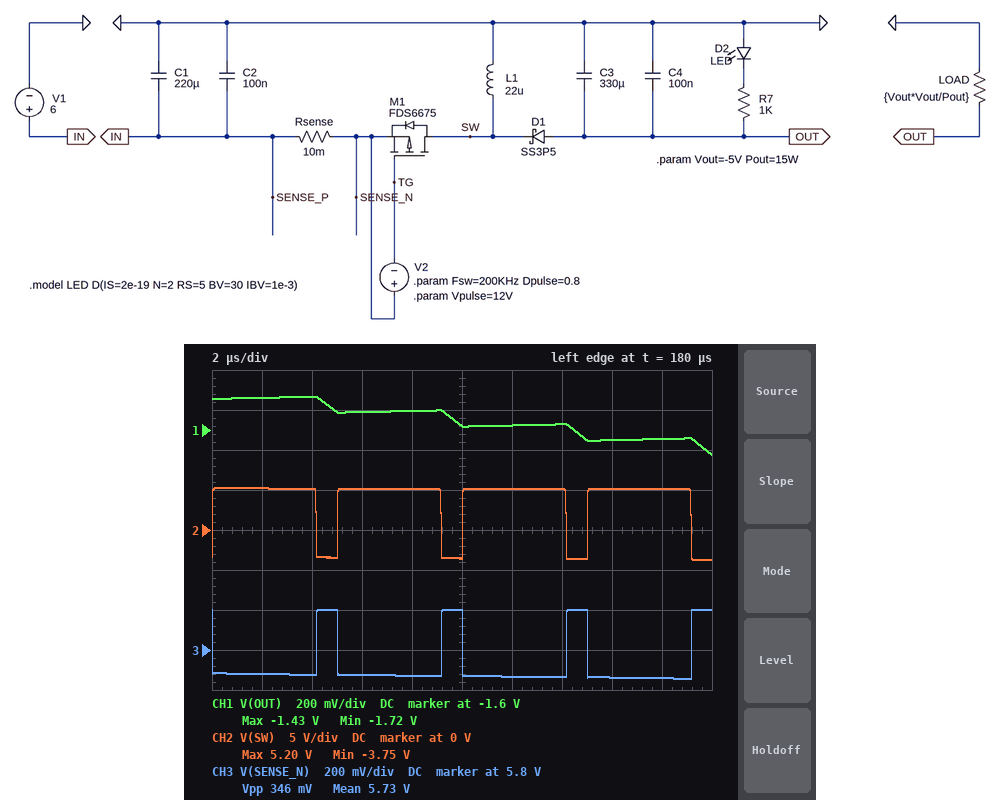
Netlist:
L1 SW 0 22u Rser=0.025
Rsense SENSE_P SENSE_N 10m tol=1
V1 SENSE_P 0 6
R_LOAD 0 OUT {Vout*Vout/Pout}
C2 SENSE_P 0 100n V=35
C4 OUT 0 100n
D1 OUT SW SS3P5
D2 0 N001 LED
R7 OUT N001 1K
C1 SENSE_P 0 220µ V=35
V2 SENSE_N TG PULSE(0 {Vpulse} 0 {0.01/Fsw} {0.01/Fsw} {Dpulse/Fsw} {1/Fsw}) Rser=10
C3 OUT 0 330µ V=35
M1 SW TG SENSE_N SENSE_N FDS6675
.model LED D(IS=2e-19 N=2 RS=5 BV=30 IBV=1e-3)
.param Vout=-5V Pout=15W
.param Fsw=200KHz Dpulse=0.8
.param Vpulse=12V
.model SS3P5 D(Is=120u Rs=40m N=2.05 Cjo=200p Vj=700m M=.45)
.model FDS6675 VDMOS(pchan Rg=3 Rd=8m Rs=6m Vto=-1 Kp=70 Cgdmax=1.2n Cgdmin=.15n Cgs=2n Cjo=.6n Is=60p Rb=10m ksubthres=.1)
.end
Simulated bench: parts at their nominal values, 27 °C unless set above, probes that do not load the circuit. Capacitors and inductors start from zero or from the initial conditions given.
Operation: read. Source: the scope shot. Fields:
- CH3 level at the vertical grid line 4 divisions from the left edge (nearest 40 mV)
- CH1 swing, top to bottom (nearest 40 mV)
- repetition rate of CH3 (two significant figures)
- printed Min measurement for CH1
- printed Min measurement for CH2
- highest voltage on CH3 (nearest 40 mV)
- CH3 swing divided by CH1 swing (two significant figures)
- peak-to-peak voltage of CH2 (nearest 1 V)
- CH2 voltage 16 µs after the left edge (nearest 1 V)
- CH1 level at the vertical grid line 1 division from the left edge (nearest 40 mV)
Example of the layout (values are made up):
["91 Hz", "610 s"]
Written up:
["5.68 V", "280 mV", "200 kHz", "-1.72 V", "-3.75 V", "6.00 V", "1.2", "9 V", "5 V", "-1.44 V"]
